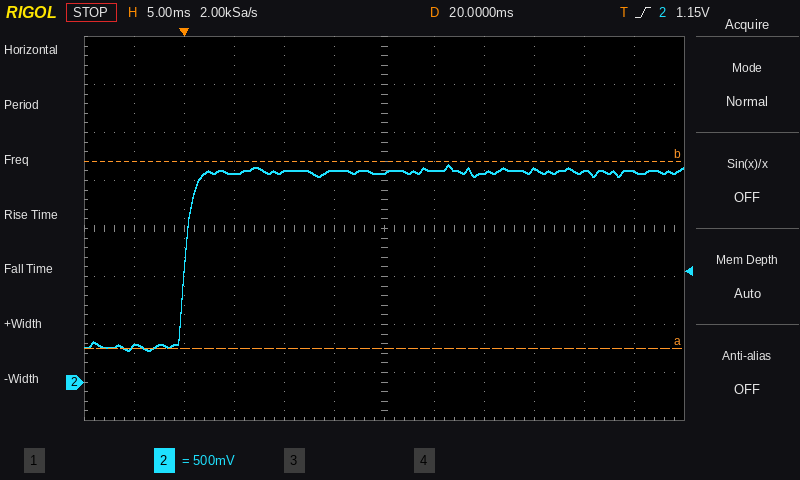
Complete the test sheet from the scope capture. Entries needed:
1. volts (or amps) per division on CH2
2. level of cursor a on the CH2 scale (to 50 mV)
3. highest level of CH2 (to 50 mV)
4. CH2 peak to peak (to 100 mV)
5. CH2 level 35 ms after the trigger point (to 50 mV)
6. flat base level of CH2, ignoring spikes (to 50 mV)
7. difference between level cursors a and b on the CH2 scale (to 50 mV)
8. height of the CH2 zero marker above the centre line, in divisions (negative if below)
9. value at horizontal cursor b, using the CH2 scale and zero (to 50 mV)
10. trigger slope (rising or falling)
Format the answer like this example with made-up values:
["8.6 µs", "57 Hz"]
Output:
["500 mV", "350 mV", "2.25 V", "1.90 V", "2.20 V", "350 mV", "1.95 V", "-3.2 div", "2.30 V", "rising"]
